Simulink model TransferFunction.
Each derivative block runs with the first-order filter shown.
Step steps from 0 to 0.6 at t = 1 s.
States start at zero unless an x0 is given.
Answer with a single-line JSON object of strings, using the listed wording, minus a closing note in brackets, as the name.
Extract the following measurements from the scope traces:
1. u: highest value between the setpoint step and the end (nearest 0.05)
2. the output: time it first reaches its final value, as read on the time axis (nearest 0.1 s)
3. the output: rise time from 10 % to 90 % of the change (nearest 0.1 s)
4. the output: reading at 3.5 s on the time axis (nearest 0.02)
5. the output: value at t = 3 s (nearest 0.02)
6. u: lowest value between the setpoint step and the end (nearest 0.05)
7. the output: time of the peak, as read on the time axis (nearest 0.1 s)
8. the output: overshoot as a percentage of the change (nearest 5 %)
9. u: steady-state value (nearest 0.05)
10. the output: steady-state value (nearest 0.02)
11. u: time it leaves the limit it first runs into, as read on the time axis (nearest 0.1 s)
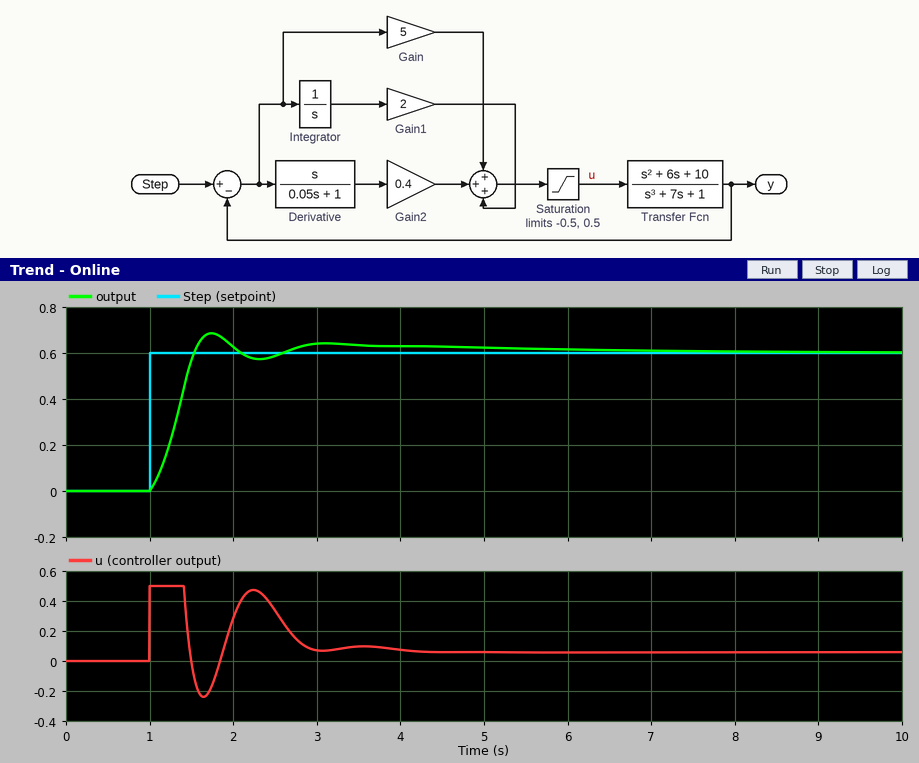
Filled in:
{"u: highest value between the setpoint step and the end": "0.50", "the output: time it first reaches its final value, as read on the time axis": "1.5 s", "the output: rise time from 10 % to 90 % of the change": "0.4 s", "the output: reading at 3.5 s on the time axis": "0.64", "the output: value at t = 3 s": "0.64", "u: lowest value between the setpoint step and the end": "-0.25", "the output: time of the peak, as read on the time axis": "1.7 s", "the output: overshoot as a percentage of the change": "15 %", "u: steady-state value": "0.05", "the output: steady-state value": "0.60", "u: time it leaves the limit it first runs into, as read on the time axis": "1.4 s"}
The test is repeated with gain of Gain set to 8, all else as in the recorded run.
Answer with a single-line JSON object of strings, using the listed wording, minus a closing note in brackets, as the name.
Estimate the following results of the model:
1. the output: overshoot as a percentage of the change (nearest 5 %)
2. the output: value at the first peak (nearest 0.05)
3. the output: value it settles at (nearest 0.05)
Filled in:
{"the output: overshoot as a percentage of the change": "10 %", "the output: value at the first peak": "0.65", "the output: value it settles at": "0.60"}
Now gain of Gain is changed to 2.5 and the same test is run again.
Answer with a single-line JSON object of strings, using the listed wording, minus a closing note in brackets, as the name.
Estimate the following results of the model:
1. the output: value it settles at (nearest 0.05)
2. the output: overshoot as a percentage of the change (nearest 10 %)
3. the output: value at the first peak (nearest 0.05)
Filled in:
{"the output: value it settles at": "0.60", "the output: overshoot as a percentage of the change": "20 %", "the output: value at the first peak": "0.70"}
